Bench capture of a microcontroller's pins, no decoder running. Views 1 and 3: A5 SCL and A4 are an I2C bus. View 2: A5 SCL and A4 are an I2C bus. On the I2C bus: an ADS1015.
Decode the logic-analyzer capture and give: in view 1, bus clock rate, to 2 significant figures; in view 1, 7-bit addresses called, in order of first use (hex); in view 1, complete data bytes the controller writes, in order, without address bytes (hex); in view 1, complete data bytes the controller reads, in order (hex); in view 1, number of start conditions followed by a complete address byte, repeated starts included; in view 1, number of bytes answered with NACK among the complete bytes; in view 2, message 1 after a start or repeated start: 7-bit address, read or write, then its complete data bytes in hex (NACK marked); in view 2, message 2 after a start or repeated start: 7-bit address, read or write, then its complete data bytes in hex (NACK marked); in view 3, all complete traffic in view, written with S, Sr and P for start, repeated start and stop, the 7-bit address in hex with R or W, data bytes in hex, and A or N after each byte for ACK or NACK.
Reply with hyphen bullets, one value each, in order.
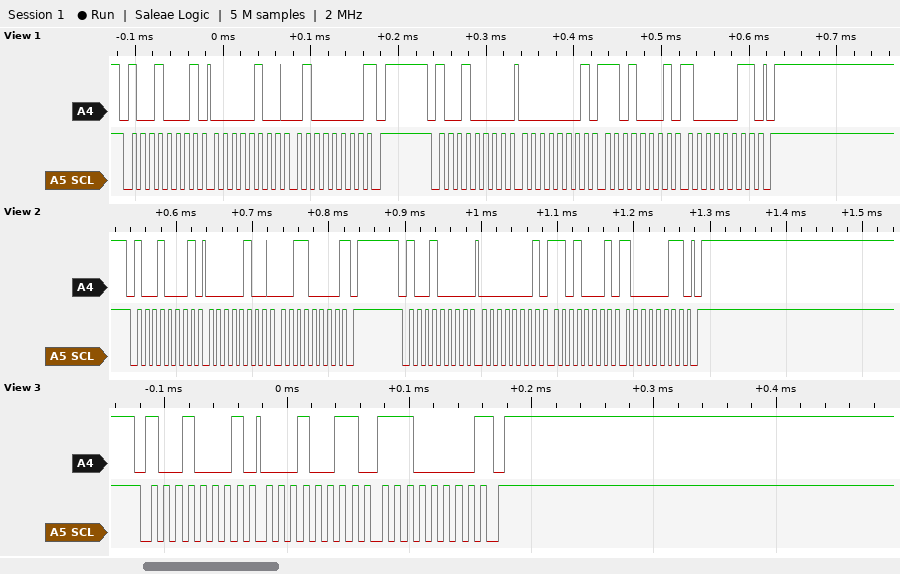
- 100 kHz
- 0x48
- 01 D1 83
- 04 40
- 2
- 1
- 0x48 read: 04 30 NACK
- 0x48 write: 01 D1 83
- S 48R A 13 A E0 N P
